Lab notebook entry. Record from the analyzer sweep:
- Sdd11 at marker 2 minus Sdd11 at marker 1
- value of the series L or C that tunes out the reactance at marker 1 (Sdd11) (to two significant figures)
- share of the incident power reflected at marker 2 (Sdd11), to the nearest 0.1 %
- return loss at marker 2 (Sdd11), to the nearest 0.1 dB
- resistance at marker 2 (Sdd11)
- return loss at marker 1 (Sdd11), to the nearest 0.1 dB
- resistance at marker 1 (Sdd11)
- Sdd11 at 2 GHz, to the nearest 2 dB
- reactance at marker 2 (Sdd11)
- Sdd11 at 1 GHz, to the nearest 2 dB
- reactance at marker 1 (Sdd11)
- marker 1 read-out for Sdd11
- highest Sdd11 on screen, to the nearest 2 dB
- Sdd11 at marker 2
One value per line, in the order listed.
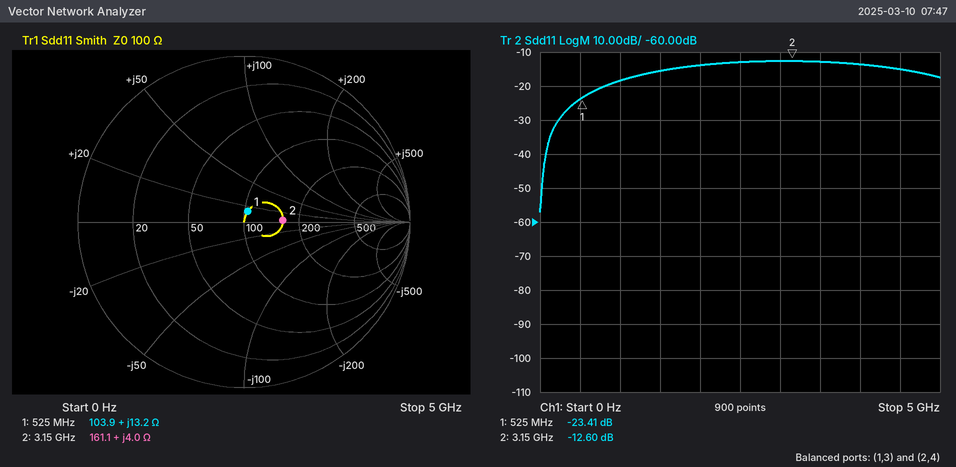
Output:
10.81 dB
23 pF
5.5 %
12.6 dB
161.1 Ω
23.4 dB
103.9 Ω
-14 dB
+4.0 Ω
-18 dB
+13.2 Ω
-23.41 dB
-12 dB
-12.60 dB
